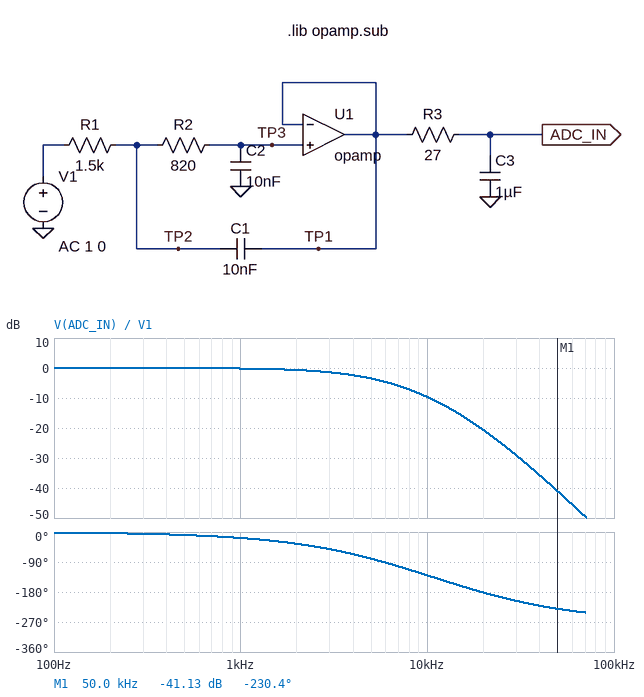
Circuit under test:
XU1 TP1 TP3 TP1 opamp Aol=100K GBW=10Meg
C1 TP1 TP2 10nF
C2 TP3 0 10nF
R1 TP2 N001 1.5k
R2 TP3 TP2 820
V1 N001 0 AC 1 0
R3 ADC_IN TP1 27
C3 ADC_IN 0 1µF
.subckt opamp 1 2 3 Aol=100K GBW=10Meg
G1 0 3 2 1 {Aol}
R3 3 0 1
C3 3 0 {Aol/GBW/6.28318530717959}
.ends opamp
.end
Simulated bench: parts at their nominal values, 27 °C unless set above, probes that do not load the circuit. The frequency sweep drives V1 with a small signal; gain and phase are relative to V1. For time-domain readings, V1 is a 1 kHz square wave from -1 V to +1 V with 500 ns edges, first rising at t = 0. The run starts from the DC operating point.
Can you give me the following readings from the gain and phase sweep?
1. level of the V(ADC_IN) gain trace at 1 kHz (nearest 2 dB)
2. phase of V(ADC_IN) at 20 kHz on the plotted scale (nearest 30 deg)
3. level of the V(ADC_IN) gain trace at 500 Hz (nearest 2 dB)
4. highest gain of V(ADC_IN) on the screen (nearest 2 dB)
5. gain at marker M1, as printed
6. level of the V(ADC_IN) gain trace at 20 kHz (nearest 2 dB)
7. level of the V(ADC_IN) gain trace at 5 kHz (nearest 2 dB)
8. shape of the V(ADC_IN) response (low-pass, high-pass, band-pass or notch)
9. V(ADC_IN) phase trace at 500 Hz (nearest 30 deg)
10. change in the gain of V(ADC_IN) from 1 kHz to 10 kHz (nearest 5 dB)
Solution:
0 dB
-180 deg
0 dB
0 dB
-41.13 dB
-20 dB
-4 dB
low-pass
0 deg
-10 dB
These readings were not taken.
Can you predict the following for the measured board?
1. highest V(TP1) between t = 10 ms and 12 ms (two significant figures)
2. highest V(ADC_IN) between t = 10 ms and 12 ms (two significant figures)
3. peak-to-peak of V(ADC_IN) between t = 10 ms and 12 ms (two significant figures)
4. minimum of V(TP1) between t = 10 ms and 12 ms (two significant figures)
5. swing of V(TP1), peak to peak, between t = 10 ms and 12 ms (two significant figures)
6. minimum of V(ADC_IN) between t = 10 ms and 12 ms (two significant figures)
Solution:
1.0 V
1.0 V
2.0 V
-1.0 V
2.0 V
-1.0 V
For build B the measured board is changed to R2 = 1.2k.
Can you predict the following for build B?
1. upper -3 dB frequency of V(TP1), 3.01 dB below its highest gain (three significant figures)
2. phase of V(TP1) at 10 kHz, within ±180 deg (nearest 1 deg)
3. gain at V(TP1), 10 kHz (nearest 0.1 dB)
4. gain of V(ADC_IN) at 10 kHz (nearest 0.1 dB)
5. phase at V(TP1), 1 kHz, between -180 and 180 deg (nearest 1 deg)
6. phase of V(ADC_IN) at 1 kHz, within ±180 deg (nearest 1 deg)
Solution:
7.57 kHz
-80 deg
-4.7 dB
-10.6 dB
-10 deg
-19 deg
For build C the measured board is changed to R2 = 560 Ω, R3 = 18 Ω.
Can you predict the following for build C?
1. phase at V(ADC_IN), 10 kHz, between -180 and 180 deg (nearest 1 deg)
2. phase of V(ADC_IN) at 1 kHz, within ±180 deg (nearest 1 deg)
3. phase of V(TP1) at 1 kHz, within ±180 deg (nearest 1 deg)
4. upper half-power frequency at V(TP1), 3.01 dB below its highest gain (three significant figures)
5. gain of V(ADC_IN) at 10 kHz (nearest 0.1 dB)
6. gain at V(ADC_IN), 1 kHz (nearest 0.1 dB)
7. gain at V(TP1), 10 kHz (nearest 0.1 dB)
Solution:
-111 deg
-14 deg
-7 deg
9.49 kHz
-6.8 dB
-0.1 dB
-3.3 dB
